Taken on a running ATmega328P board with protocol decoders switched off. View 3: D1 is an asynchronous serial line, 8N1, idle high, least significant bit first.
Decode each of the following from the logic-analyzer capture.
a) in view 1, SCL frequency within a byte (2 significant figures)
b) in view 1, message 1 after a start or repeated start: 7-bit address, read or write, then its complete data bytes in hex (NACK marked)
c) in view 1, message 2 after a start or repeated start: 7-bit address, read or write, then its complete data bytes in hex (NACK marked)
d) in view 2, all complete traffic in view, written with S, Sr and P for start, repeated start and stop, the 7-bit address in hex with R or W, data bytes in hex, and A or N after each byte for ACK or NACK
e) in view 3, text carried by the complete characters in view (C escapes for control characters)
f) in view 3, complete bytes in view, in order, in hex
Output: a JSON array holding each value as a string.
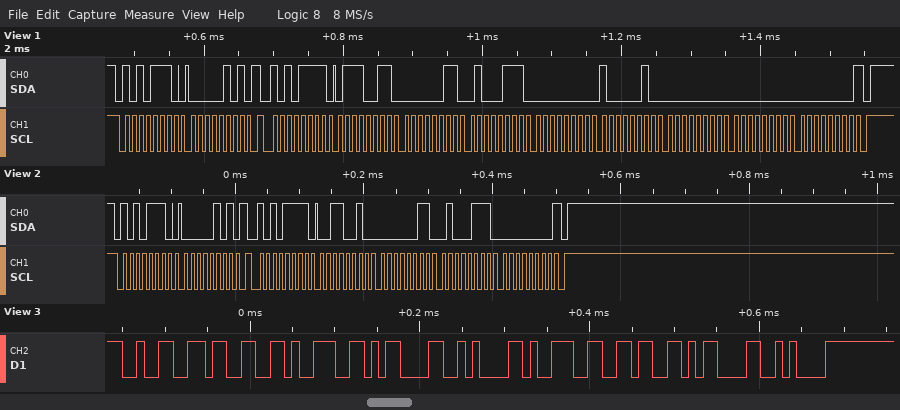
["100 kHz", "0x57 write: 05", "0x57 read: 73 03 47 00 82 00 00 00 NACK", "S 57W A 05 A Sr 57R A 32 A 03 A 47 A 00 N P", "\"239\\r\\n96\\r\\n\"", "32 33 39 0D 0A 39 36 0D 0A"]
